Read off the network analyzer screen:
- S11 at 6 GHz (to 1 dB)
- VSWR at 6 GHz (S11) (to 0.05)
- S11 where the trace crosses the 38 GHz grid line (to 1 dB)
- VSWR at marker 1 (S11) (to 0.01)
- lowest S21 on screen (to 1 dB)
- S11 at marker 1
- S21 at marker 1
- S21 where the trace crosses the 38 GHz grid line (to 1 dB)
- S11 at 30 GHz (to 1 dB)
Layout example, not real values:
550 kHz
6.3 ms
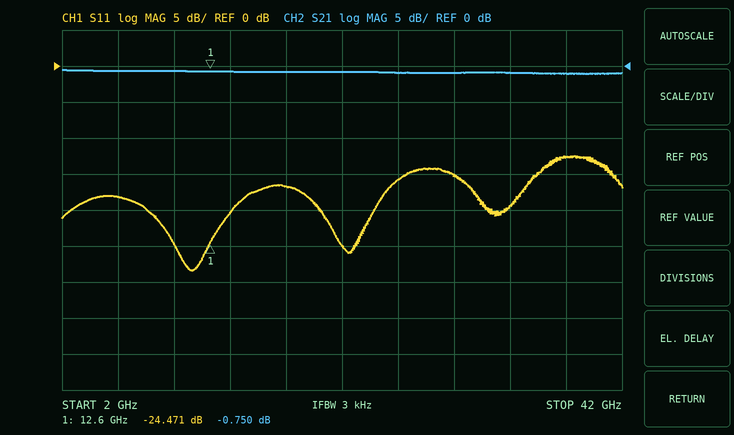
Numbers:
-18 dB
1.30
-13 dB
1.13
-1 dB
-24.471 dB
-0.750 dB
-1 dB
-15 dB
